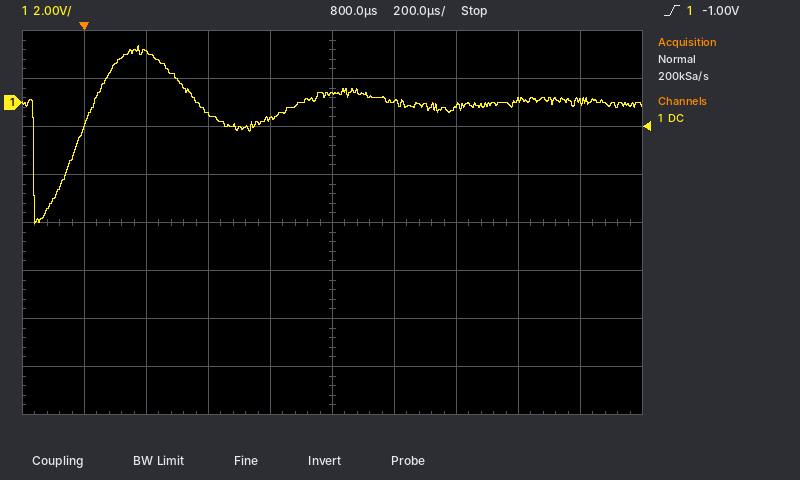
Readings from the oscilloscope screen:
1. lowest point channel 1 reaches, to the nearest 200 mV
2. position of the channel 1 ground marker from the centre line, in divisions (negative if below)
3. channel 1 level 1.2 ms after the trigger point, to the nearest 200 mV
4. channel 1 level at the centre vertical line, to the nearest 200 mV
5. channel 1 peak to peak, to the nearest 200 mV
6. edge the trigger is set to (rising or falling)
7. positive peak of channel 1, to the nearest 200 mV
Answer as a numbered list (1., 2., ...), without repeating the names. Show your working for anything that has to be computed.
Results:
1. -5.0 V
2. +2.5 div
3. -200 mV
4. 400 mV
5. 2.4 V − (-5.0 V) = 7.4 V
6. rising
7. 2.4 V
